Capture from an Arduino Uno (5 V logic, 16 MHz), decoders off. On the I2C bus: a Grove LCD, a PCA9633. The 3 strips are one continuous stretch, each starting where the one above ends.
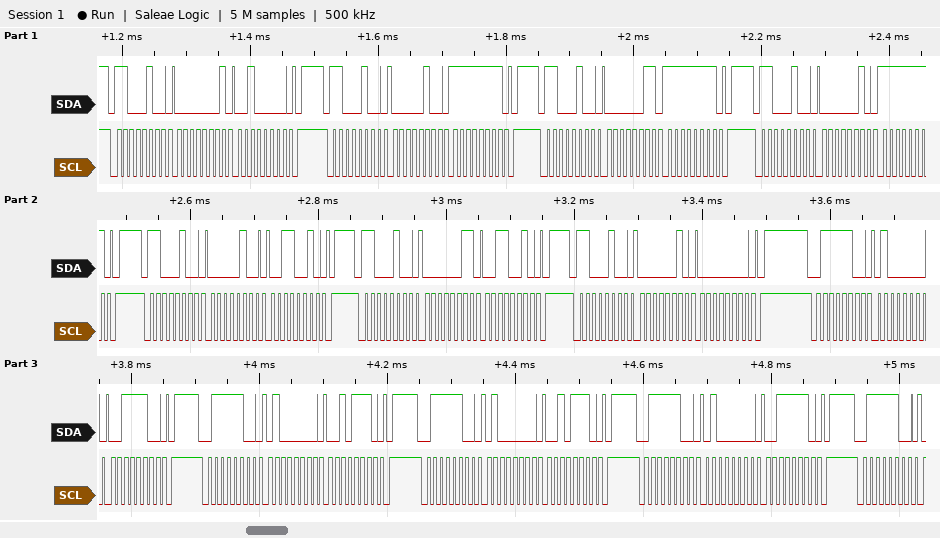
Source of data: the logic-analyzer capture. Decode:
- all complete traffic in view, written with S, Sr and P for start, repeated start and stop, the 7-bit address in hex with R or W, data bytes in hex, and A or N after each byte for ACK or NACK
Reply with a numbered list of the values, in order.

1. S 62W A 01 A 20 A P S 62W A 04 A FF A P S 62W A 03 A FF A P S 62W A 02 A FF A P S 62W A 04 A 32 A P S 62W A 03 A 32 A P S 62W A 02 A 00 A P S 3EW A 40 A 3C A P S 3EW A 40 A 2E A P S 3EW A 40 A 2E A P S 3EW A 40 A 3E A P S 3EW A
